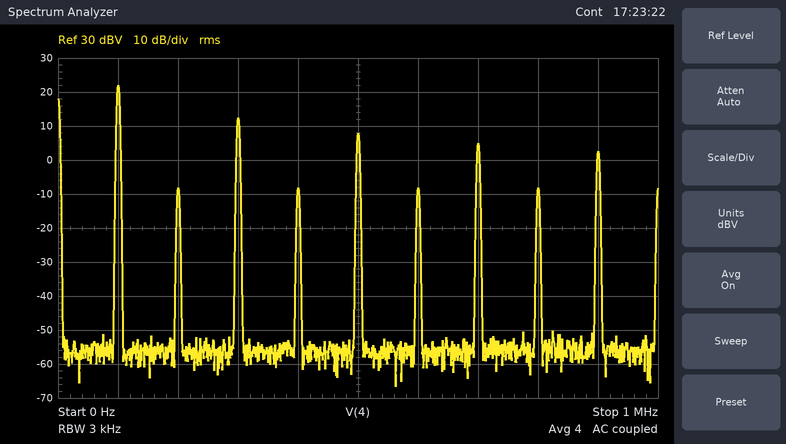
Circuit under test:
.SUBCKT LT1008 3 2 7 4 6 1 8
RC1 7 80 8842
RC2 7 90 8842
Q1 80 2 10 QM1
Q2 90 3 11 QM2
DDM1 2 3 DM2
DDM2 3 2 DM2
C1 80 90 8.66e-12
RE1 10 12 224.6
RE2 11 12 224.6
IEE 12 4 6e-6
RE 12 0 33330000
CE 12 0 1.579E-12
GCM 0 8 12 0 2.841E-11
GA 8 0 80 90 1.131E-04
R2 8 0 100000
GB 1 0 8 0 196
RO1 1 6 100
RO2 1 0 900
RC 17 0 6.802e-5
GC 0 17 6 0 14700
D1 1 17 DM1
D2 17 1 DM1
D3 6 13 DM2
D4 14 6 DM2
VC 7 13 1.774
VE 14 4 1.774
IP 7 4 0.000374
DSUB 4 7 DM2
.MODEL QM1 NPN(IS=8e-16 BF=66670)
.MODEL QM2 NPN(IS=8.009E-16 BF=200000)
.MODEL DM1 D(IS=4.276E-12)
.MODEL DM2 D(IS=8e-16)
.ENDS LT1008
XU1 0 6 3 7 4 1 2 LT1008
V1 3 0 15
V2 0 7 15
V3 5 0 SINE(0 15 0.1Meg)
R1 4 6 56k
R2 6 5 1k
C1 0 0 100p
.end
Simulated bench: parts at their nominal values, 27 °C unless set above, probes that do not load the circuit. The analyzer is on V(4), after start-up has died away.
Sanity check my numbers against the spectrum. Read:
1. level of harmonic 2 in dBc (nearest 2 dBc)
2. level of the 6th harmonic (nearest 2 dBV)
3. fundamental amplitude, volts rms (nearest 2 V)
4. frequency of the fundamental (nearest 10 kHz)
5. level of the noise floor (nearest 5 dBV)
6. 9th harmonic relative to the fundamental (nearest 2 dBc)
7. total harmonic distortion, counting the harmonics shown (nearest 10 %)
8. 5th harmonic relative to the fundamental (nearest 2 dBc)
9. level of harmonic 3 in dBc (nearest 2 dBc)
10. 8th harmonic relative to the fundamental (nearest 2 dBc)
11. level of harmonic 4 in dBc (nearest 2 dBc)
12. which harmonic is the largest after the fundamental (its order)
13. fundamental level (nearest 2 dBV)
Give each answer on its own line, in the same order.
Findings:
-30 dBc
-8 dBV
12 V
100 kHz
-55 dBV
-20 dBc
40 %
-14 dBc
-10 dBc
-30 dBc
-30 dBc
3
22 dBV
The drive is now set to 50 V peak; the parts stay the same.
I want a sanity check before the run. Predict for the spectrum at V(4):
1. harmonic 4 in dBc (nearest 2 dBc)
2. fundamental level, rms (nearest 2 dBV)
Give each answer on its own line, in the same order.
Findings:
-26 dBc
22 dBV
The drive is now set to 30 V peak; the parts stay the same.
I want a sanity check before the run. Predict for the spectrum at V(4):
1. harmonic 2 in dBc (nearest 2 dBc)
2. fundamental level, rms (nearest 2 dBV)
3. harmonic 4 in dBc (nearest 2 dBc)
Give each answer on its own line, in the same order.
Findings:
-26 dBc
22 dBV
-26 dBc
